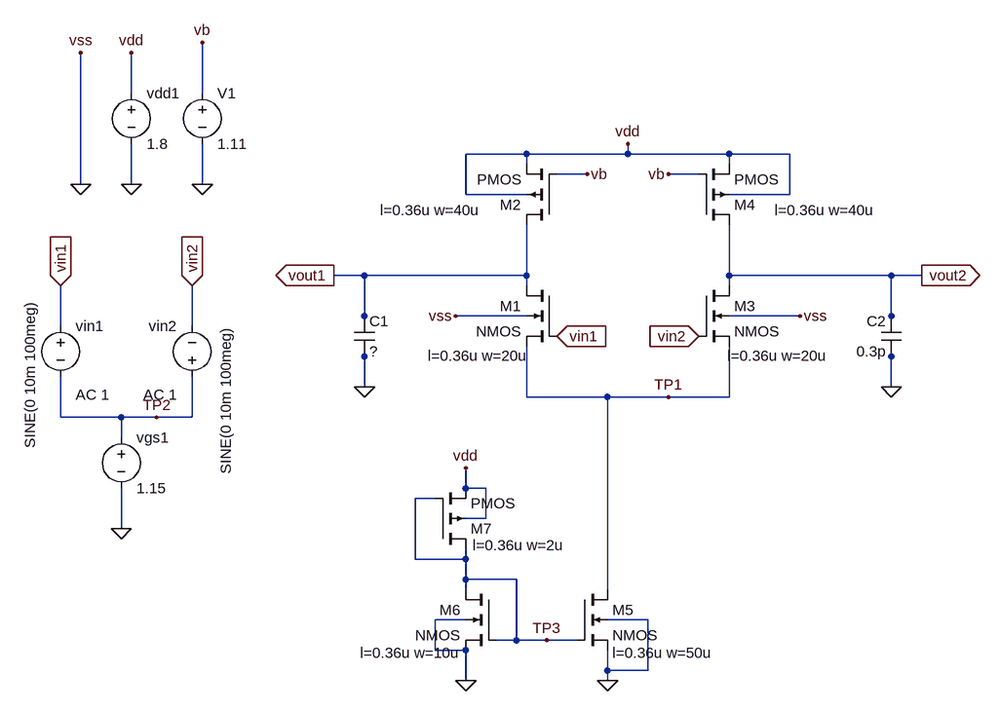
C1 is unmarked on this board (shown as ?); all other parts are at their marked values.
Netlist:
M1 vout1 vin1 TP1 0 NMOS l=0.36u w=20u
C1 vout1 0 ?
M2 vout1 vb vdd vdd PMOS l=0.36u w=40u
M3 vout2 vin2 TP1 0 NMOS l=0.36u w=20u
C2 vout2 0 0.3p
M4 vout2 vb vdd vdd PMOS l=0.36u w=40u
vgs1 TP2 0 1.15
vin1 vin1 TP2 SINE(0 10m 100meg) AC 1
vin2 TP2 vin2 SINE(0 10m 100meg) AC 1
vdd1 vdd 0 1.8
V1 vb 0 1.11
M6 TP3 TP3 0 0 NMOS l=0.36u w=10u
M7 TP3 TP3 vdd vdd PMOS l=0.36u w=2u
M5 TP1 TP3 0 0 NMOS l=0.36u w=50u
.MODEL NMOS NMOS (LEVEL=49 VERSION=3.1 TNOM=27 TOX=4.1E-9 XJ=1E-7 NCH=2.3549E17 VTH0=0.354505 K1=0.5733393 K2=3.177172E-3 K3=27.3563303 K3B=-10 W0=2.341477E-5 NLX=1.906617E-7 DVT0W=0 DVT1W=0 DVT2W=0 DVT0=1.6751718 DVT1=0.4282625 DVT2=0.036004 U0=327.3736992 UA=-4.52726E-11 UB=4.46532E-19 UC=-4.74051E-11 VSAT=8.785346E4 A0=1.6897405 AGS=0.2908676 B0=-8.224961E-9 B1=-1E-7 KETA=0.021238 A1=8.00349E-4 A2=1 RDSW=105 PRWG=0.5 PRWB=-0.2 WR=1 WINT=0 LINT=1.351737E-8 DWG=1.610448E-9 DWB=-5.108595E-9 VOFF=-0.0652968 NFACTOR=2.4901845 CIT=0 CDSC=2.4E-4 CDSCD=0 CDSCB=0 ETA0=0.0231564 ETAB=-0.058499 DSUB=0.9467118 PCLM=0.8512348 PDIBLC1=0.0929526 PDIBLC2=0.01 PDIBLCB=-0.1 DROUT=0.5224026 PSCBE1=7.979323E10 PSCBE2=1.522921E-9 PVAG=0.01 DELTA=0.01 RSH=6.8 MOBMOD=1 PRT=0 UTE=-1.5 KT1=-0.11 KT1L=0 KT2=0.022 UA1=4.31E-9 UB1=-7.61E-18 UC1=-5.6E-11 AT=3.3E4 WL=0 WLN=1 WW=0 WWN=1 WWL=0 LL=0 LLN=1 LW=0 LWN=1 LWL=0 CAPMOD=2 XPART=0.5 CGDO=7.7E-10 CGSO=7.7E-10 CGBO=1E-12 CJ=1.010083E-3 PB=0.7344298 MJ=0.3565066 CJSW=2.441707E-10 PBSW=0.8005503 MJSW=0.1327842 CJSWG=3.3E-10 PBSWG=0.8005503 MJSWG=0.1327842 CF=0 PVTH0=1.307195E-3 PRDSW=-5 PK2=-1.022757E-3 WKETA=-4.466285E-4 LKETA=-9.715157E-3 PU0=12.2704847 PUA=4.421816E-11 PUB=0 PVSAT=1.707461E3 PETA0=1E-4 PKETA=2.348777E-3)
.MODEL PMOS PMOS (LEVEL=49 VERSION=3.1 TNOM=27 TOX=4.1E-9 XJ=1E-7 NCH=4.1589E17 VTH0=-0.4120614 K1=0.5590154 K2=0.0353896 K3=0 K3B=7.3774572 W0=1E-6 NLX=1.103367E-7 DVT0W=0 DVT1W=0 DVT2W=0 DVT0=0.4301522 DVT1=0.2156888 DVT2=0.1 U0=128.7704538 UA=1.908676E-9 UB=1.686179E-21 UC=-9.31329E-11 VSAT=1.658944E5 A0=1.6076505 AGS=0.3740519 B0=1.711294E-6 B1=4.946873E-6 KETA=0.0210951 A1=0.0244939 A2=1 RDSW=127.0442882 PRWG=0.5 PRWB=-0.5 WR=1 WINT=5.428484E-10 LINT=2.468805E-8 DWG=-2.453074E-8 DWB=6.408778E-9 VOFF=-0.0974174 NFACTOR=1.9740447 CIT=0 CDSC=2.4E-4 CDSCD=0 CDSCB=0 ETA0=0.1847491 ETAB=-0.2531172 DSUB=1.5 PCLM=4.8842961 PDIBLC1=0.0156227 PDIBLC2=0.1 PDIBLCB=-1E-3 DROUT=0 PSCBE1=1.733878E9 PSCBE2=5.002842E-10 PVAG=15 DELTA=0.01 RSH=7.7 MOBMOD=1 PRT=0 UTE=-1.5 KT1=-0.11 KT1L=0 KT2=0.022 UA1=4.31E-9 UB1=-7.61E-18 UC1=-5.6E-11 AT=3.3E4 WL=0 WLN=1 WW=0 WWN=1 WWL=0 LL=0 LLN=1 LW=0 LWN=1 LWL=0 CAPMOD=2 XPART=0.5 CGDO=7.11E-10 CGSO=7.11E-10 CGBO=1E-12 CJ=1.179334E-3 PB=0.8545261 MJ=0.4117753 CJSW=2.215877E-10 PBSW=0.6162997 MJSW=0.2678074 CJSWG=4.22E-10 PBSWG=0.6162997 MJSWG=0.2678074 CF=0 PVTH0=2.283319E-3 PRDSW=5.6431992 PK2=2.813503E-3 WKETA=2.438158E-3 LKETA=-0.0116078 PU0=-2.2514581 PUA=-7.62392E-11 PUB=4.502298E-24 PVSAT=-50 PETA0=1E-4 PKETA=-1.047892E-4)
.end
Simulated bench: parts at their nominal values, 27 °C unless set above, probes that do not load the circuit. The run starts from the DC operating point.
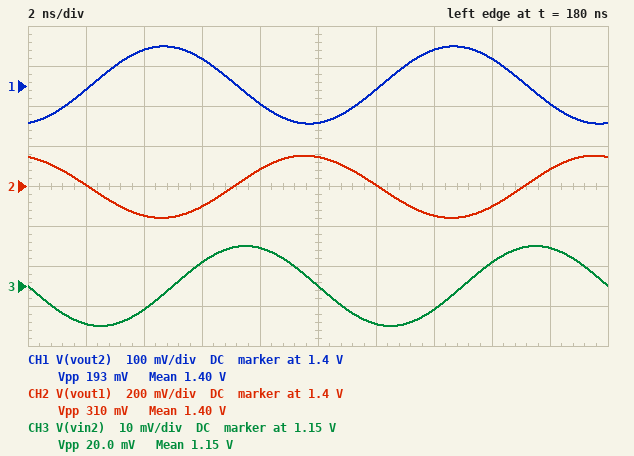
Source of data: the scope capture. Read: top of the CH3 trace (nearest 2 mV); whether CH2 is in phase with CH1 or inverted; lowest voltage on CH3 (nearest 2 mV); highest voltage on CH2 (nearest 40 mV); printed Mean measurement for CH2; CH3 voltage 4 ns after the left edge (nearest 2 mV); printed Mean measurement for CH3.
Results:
1.160 V
inverted
1.140 V
1.56 V
1.40 V
1.144 V
1.15 V
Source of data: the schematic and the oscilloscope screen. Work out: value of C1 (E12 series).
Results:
180 fF
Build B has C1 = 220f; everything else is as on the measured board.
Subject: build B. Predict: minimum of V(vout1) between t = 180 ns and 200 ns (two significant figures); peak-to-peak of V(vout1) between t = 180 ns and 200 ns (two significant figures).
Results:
1.3 V
270 mV
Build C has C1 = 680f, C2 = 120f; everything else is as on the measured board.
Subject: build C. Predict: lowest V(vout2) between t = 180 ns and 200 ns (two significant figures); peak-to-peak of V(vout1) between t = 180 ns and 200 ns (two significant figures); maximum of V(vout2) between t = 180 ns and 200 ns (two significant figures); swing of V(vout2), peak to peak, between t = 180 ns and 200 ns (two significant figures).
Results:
1.2 V
98 mV
1.6 V
370 mV
